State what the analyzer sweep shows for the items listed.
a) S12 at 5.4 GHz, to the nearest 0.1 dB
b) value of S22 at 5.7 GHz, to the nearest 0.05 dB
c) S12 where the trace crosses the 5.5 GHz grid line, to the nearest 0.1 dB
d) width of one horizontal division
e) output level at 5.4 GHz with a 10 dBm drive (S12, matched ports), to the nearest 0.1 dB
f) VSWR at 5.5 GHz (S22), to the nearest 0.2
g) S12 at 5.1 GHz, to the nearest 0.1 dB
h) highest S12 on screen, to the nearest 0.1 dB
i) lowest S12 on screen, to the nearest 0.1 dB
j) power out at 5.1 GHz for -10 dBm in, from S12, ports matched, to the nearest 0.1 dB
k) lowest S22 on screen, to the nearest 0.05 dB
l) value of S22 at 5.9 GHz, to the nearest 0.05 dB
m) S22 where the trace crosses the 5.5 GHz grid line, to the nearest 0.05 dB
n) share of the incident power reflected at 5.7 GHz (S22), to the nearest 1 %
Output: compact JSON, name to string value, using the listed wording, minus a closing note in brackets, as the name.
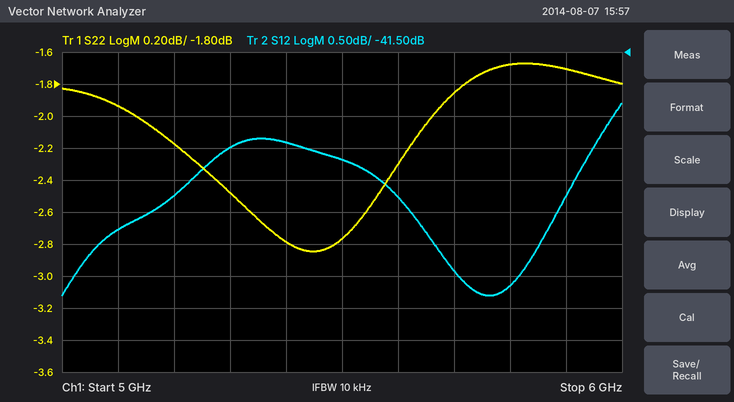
{"S12 at 5.4 GHz, to the nearest 0.1 dB": "-42.9 dB", "value of S22 at 5.7 GHz, to the nearest 0.05 dB": "-1.85 dB", "S12 where the trace crosses the 5.5 GHz grid line, to the nearest 0.1 dB": "-43.2 dB", "width of one horizontal division": "100 MHz", "output level at 5.4 GHz with a 10 dBm drive (S12, matched ports), to the nearest 0.1 dB": "-32.9 dBm", "VSWR at 5.5 GHz (S22), to the nearest 0.2": "6.4", "S12 at 5.1 GHz, to the nearest 0.1 dB": "-44.3 dB", "highest S12 on screen, to the nearest 0.1 dB": "-42.3 dB", "lowest S12 on screen, to the nearest 0.1 dB": "-45.3 dB", "power out at 5.1 GHz for -10 dBm in, from S12, ports matched, to the nearest 0.1 dB": "-54.3 dBm", "lowest S22 on screen, to the nearest 0.05 dB": "-2.85 dB", "value of S22 at 5.9 GHz, to the nearest 0.05 dB": "-1.70 dB", "S22 where the trace crosses the 5.5 GHz grid line, to the nearest 0.05 dB": "-2.75 dB", "share of the incident power reflected at 5.7 GHz (S22), to the nearest 1 %": "65 %"}
